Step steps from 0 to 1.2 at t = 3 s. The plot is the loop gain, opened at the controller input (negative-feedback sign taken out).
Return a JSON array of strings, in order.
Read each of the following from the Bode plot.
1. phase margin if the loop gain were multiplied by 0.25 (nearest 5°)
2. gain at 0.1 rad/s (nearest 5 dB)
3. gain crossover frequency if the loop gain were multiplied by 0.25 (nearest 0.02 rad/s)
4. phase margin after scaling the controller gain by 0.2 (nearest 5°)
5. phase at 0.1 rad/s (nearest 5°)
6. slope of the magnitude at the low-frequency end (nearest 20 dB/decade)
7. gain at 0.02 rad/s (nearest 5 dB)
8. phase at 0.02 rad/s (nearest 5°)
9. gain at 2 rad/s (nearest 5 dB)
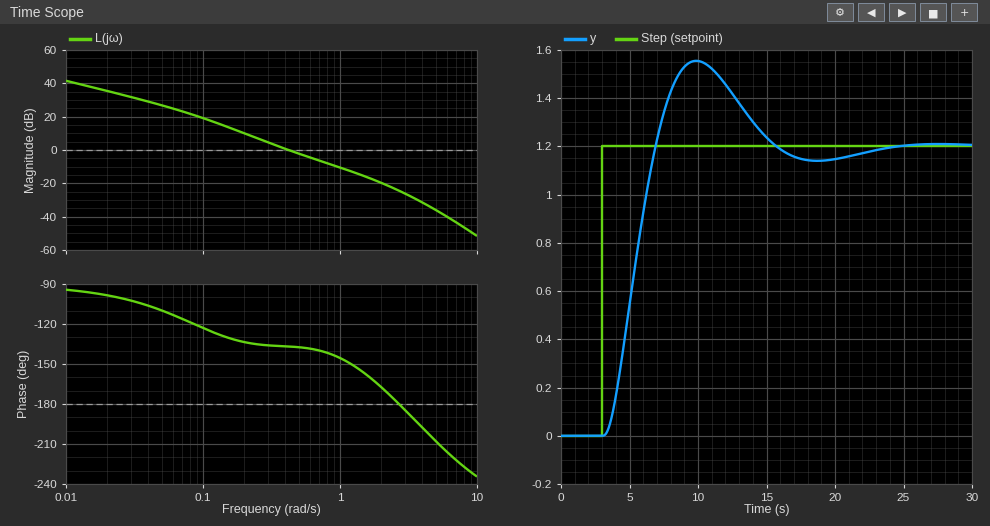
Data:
["50°", "20 dB", "0.18 rad/s", "50°", "-125°", "-20 dB/decade", "35 dB", "-100°", "-20 dB"]
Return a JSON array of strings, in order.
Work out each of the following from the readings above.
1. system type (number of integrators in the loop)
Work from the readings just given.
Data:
["1"]
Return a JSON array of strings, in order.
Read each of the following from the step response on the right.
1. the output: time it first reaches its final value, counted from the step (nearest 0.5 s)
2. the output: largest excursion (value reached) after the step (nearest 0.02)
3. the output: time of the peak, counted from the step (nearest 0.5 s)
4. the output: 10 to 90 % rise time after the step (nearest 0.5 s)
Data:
["4.0 s", "1.56", "7.0 s", "2.5 s"]
